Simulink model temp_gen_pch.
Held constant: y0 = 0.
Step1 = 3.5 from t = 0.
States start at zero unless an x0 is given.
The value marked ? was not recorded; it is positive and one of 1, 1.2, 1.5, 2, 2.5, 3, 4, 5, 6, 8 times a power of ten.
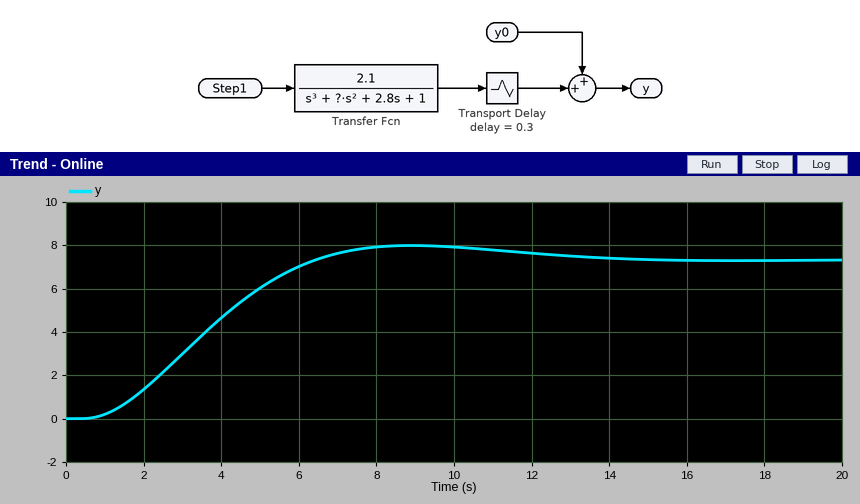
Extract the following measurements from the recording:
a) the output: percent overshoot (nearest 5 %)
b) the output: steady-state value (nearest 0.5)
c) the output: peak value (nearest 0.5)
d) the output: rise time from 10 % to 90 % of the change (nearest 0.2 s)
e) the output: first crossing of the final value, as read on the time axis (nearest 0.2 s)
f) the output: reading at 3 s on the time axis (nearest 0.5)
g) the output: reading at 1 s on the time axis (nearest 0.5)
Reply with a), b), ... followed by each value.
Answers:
a) 10 %
b) 7.5
c) 8.0
d) 4.0 s
e) 6.4 s
f) 3.0
g) 0.0
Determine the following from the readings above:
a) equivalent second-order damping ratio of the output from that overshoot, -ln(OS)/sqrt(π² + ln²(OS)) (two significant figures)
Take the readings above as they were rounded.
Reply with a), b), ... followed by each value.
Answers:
a) 0.59
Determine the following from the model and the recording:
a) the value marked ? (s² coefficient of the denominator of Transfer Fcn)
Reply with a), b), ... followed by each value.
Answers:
a) 5
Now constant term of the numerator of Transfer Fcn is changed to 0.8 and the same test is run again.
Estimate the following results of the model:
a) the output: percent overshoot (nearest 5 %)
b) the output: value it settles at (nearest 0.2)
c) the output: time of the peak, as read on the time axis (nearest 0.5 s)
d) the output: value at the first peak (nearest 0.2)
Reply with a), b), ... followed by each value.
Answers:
a) 10 %
b) 2.8
c) 9.0 s
d) 3.0
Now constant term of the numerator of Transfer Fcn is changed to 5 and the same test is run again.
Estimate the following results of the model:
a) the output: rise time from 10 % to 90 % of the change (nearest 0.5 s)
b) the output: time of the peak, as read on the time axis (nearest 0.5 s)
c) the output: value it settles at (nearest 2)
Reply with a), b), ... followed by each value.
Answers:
a) 4.0 s
b) 9.0 s
c) 18
